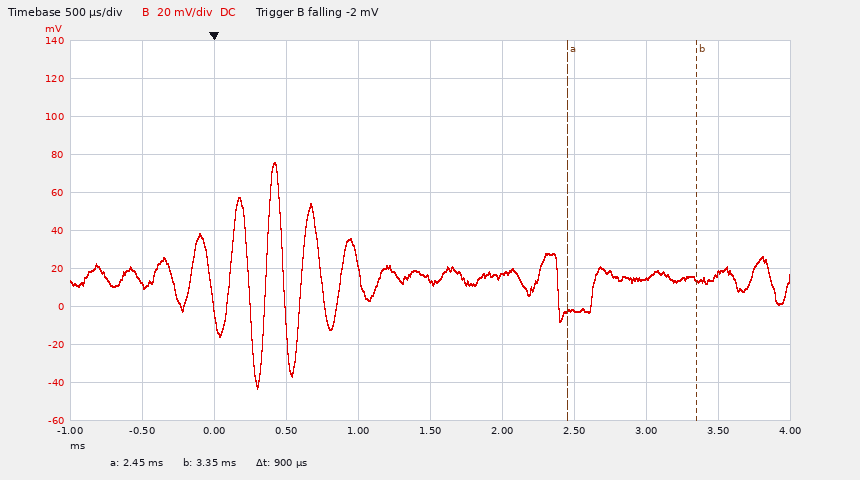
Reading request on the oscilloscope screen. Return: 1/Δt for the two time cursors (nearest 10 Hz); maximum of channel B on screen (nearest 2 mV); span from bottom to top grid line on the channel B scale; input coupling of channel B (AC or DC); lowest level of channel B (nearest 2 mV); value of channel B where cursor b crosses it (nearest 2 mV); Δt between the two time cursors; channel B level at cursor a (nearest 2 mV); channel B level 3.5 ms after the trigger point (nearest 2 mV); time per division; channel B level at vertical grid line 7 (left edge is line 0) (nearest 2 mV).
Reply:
1.11 kHz
76 mV
200 mV
DC
-44 mV
14 mV
900 µs
-2 mV
18 mV
500 µs
-2 mV
